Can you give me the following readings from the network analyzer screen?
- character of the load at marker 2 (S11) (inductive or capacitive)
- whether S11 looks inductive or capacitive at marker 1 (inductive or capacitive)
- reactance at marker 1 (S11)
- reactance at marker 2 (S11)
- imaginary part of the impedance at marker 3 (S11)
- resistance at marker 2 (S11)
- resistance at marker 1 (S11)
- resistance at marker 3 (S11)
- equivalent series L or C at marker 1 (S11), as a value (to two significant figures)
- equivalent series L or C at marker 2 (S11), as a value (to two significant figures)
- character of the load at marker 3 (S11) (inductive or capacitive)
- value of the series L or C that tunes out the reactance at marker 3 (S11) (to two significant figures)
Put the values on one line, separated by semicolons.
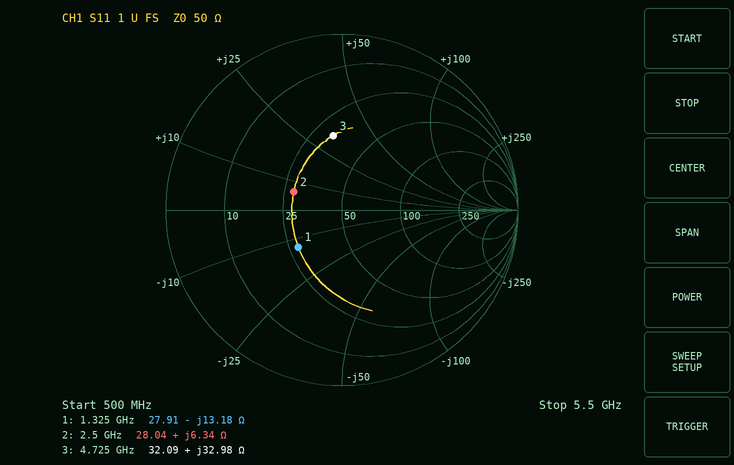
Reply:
inductive; capacitive; -13.18 Ω; +6.34 Ω; +32.98 Ω; 28.04 Ω; 27.91 Ω; 32.09 Ω; 9.1 pF; 400 pH; inductive; 1.0 pF
